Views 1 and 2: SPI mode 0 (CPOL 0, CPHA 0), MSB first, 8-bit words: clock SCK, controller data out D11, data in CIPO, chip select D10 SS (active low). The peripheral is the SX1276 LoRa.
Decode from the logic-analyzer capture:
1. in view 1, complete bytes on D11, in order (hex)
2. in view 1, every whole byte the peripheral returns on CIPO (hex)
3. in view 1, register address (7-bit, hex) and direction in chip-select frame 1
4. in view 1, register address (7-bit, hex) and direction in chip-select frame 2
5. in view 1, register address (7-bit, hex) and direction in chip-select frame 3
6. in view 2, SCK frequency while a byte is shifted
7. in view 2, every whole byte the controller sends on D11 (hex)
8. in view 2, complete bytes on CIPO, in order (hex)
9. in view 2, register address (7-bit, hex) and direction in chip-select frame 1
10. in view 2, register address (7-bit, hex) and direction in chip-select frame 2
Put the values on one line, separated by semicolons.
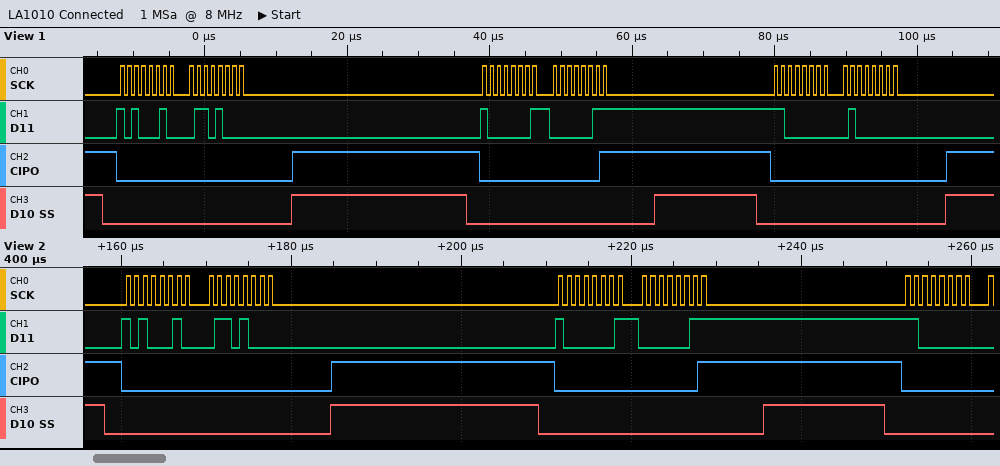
0xA2 0x68 0x81 0x03 0xC0 0x40; 0x00 0x00 0x00 0x01 0x00 0x00; 0x22 write; 0x01 write; 0x40 write; 1 MHz; A2 68 81 03 C0; 00 00 00 01 00; 0x22 write; 0x01 write
